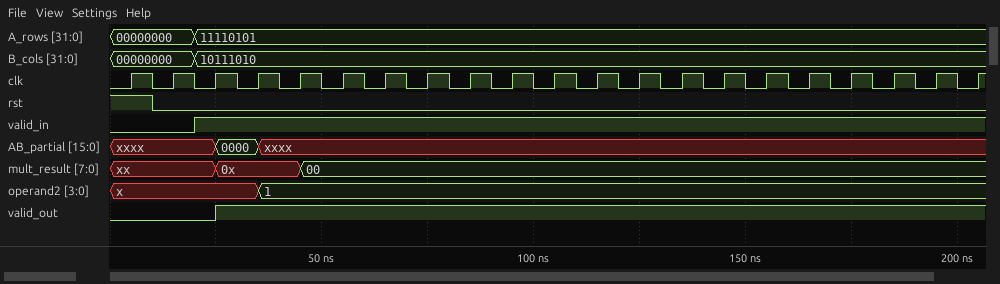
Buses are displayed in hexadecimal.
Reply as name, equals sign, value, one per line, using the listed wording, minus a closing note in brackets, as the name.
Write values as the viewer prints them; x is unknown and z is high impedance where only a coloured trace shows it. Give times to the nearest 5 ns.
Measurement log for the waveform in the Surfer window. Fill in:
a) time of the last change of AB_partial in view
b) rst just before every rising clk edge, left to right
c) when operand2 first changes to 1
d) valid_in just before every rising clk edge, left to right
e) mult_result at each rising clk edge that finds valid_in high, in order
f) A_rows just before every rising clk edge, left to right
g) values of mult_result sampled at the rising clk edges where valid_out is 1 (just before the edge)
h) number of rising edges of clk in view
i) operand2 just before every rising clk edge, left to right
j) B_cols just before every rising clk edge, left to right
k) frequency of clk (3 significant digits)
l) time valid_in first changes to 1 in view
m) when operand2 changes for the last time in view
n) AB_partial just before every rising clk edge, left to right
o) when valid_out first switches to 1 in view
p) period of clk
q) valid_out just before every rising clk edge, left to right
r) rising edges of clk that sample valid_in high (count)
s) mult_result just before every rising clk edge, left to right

time of the last change of AB_partial in view = 35 ns
rst just before every rising clk edge, left to right = 1 0 0 0 0 0 0 0 0 0 0 0 0 0 0 0 0 0 0 0 0
when operand2 first changes to 1 = 35 ns
valid_in just before every rising clk edge, left to right = 0 0 1 1 1 1 1 1 1 1 1 1 1 1 1 1 1 1 1 1 1
mult_result at each rising clk edge that finds valid_in high, in order = xx, 0x, 0x, 00, 00, 00, 00, 00, 00, 00, 00, 00, 00, 00, 00, 00, 00, 00, 00
A_rows just before every rising clk edge, left to right = 00000000, 00000000, 11110101, 11110101, 11110101, 11110101, 11110101, 11110101, 11110101, 11110101, 11110101, 11110101, 11110101, 11110101, 11110101, 11110101, 11110101, 11110101, 11110101, 11110101, 11110101
values of mult_result sampled at the rising clk edges where valid_out is 1 = 0x, 0x, 00, 00, 00, 00, 00, 00, 00, 00, 00, 00, 00, 00, 00, 00, 00, 00
number of rising edges of clk in view = 21
operand2 just before every rising clk edge, left to right = x, x, x, x, 1, 1, 1, 1, 1, 1, 1, 1, 1, 1, 1, 1, 1, 1, 1, 1, 1
B_cols just before every rising clk edge, left to right = 00000000, 00000000, 10111010, 10111010, 10111010, 10111010, 10111010, 10111010, 10111010, 10111010, 10111010, 10111010, 10111010, 10111010, 10111010, 10111010, 10111010, 10111010, 10111010, 10111010, 10111010
frequency of clk = 100 MHz
time valid_in first changes to 1 in view = 20 ns
when operand2 changes for the last time in view = 35 ns
AB_partial just before every rising clk edge, left to right = xxxx, xxxx, xxxx, 0000, xxxx, xxxx, xxxx, xxxx, xxxx, xxxx, xxxx, xxxx, xxxx, xxxx, xxxx, xxxx, xxxx, xxxx, xxxx, xxxx, xxxx
when valid_out first switches to 1 in view = 25 ns
period of clk = 10 ns
valid_out just before every rising clk edge, left to right = 0 0 0 1 1 1 1 1 1 1 1 1 1 1 1 1 1 1 1 1 1
rising edges of clk that sample valid_in high = 19
mult_result just before every rising clk edge, left to right = xx, xx, xx, 0x, 0x, 00, 00, 00, 00, 00, 00, 00, 00, 00, 00, 00, 00, 00, 00, 00, 00
